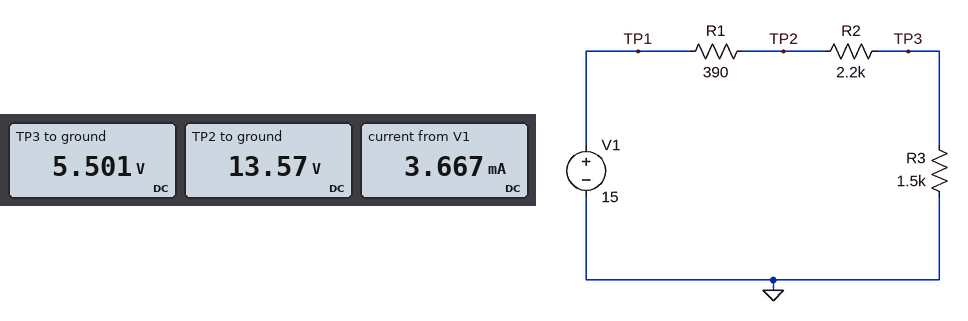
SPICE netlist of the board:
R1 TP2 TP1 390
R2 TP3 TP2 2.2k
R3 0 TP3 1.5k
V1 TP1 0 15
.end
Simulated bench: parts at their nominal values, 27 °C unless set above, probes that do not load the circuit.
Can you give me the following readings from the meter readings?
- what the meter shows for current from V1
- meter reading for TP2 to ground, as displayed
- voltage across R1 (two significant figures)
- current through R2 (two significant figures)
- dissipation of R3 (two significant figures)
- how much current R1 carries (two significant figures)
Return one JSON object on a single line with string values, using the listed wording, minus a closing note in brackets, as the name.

{"what the meter shows for current from V1": "3.667 mA", "meter reading for TP2 to ground, as displayed": "13.57 V", "voltage across R1": "1.4 V", "current through R2": "3.7 mA", "dissipation of R3": "20 mW", "how much current R1 carries": "3.7 mA"}
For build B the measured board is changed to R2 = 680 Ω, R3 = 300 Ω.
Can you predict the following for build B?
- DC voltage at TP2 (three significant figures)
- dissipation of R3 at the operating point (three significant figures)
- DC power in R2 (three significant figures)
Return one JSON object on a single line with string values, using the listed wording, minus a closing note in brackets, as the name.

{"DC voltage at TP2": "10.7 V", "dissipation of R3 at the operating point": "36.0 mW", "DC power in R2": "81.5 mW"}
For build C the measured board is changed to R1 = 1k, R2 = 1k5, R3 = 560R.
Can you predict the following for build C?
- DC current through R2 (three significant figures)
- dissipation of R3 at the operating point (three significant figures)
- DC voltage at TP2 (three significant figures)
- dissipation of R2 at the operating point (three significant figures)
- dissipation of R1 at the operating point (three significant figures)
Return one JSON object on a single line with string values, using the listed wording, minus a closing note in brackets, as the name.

{"DC current through R2": "4.90 mA", "dissipation of R3 at the operating point": "13.5 mW", "DC voltage at TP2": "10.1 V", "dissipation of R2 at the operating point": "36.0 mW", "dissipation of R1 at the operating point": "24.0 mW"}
